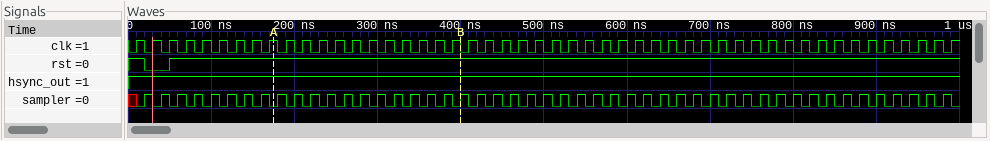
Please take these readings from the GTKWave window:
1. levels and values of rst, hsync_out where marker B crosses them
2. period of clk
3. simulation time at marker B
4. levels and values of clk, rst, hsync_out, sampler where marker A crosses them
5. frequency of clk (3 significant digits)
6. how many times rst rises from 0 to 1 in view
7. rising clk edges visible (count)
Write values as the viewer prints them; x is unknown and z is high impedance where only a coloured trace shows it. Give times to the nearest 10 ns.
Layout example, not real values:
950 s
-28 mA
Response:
rst=1, hsync_out=1
20 ns
400 ns
clk=1, rst=1, hsync_out=1, sampler=0
50.0 MHz
1
50
